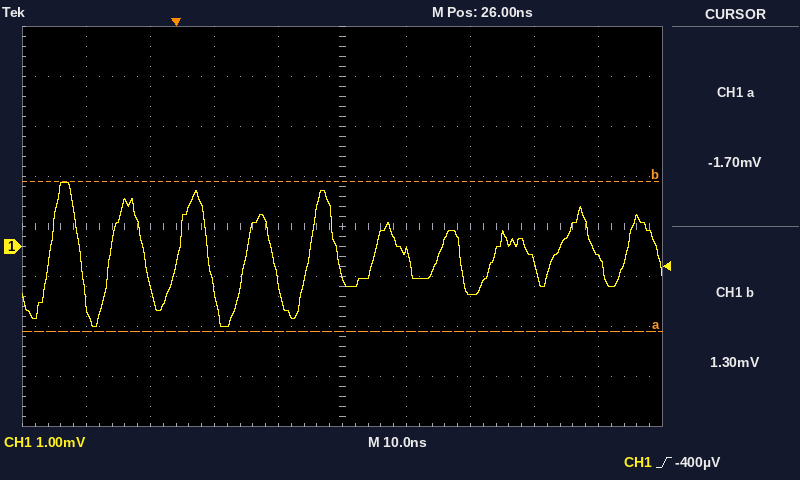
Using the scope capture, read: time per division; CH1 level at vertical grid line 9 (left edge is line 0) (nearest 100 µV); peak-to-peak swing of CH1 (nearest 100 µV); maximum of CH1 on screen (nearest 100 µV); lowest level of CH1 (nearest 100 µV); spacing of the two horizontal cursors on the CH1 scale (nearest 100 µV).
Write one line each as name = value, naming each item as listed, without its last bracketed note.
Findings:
time per division = 10 ns
CH1 level at vertical grid line 9 (left edge is line 0) = -200 µV
peak-to-peak swing of CH1 = 2.9 mV
maximum of CH1 on screen = 1.3 mV
lowest level of CH1 = -1.6 mV
spacing of the two horizontal cursors on the CH1 scale = 3.0 mV
